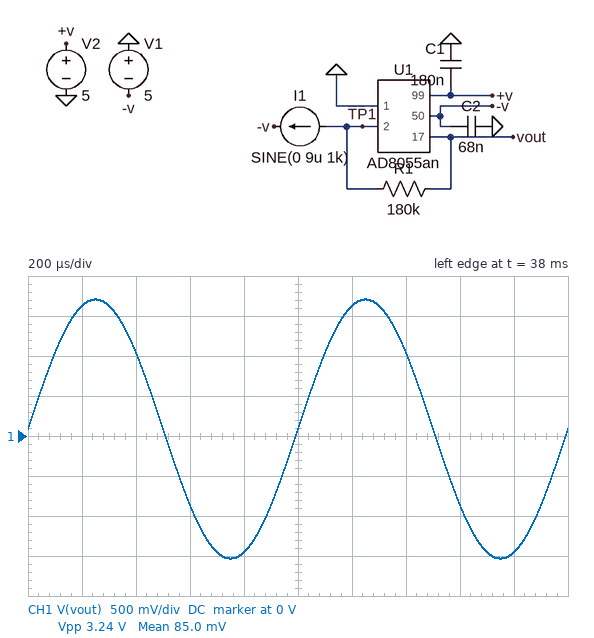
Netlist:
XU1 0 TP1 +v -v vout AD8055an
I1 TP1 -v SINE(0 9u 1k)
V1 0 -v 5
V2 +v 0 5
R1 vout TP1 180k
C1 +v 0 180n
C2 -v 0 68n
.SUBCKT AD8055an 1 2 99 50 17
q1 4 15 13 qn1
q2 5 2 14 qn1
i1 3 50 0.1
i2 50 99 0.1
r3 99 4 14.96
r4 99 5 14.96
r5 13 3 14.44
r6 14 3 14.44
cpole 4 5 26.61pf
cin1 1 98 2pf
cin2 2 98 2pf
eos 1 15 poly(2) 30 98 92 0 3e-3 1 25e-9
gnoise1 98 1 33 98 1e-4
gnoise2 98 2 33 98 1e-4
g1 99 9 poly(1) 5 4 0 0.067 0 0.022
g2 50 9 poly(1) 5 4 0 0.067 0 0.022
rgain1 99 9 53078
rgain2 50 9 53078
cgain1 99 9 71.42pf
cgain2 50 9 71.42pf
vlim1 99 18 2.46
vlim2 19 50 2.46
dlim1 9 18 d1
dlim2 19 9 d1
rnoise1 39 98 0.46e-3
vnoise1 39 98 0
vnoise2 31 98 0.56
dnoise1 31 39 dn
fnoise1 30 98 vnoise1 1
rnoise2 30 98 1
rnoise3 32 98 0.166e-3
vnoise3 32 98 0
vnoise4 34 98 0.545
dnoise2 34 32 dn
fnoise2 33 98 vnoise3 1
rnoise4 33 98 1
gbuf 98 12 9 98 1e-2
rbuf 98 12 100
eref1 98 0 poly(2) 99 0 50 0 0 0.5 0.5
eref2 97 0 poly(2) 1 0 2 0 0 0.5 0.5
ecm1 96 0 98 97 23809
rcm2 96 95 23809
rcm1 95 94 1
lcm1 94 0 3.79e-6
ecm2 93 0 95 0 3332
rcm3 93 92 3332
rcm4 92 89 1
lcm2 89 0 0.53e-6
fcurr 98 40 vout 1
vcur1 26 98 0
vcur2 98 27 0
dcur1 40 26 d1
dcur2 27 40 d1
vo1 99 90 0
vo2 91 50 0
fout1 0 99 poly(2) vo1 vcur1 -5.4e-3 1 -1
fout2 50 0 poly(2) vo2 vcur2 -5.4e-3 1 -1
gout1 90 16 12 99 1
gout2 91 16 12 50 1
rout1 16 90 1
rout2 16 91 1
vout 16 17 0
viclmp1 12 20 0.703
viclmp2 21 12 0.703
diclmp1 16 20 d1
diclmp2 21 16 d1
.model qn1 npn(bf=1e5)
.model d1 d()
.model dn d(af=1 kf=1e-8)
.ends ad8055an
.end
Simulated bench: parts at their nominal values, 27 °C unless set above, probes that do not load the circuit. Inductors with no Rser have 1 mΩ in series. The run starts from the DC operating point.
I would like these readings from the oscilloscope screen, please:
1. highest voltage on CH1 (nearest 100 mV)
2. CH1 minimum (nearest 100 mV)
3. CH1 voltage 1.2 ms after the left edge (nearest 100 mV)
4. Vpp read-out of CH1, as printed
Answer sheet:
1.7 V
-1.5 V
1.6 V
3.24 V
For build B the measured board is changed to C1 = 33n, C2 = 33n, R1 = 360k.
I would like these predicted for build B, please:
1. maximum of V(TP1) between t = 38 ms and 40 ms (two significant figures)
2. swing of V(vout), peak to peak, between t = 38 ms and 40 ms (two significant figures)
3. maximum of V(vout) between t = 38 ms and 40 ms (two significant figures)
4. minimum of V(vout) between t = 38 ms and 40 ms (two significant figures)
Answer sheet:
-2.1 mV
6.3 V
3.3 V
-3.1 V
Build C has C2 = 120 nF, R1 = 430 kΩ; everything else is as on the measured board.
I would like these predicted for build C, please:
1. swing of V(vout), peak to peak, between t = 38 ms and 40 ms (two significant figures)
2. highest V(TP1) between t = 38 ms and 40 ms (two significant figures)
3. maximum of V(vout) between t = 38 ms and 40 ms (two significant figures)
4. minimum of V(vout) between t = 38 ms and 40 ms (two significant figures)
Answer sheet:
6.6 V
320 mV
3.3 V
-3.3 V
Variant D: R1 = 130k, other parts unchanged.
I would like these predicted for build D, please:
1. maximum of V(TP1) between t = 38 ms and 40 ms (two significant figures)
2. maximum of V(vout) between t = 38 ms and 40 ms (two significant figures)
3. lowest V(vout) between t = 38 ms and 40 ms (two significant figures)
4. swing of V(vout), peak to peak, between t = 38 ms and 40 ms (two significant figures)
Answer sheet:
-2.7 mV
1.2 V
-1.1 V
2.3 V
